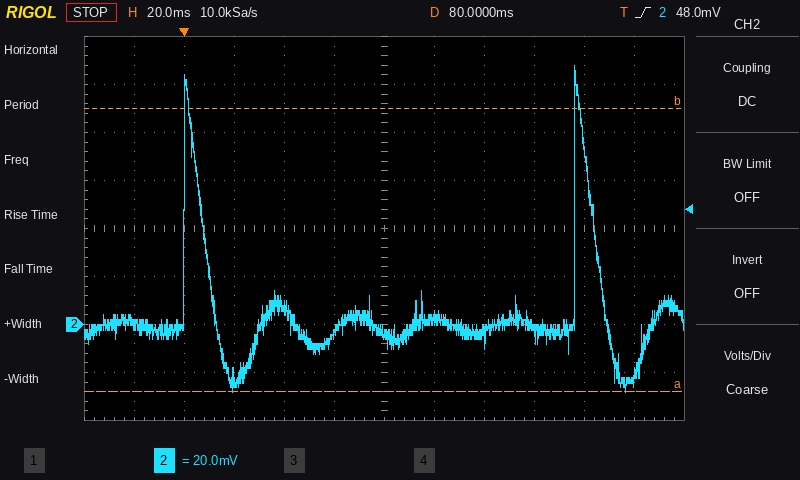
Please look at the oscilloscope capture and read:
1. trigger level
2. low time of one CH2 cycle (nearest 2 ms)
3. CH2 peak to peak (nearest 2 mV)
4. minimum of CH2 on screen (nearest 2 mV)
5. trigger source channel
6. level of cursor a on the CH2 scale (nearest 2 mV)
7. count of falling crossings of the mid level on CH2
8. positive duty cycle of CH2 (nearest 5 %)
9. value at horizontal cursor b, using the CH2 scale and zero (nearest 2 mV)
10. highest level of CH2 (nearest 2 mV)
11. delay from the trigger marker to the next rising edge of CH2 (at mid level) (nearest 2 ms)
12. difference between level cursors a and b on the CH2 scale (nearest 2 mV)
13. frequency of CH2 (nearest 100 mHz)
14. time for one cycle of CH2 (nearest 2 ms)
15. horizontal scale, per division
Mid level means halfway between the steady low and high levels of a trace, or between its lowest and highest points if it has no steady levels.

48.0 mV
148 ms
136 mV
-28 mV
CH2
-28 mV
2
5 %
90 mV
108 mV
156 ms
118 mV
6.4 Hz
156 ms
20 ms
